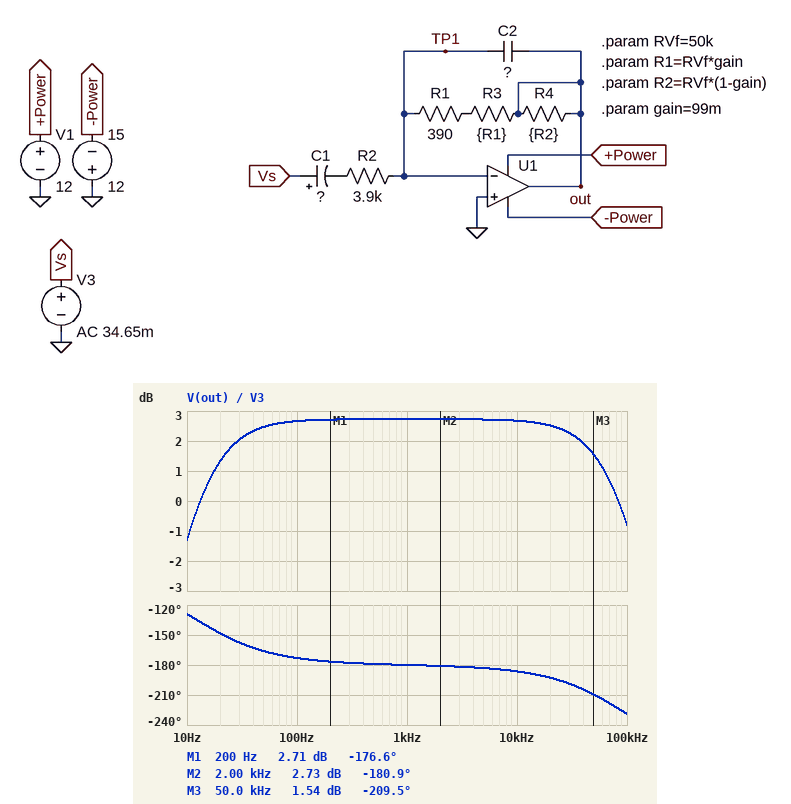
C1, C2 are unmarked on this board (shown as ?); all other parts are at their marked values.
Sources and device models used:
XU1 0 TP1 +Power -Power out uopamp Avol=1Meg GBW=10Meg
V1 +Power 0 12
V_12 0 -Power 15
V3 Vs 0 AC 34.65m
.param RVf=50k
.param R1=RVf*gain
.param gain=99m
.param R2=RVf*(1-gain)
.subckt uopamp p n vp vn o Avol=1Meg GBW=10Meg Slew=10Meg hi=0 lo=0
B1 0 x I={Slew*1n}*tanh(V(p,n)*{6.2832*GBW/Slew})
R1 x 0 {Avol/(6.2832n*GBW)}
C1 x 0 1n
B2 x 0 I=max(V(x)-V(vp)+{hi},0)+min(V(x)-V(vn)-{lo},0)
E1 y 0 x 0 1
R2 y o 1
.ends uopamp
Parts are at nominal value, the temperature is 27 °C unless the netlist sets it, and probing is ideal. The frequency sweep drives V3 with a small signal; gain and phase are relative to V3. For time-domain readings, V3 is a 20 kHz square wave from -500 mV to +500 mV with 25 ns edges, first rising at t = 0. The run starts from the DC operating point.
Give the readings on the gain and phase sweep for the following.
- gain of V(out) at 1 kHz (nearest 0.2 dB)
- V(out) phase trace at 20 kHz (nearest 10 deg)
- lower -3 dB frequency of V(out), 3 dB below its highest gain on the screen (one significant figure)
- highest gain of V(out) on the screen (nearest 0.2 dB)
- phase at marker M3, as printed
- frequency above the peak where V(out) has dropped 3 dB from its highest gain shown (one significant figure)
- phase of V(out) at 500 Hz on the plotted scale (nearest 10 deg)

2.8 dB
-190 deg
10 Hz
2.8 dB
-209.5 deg
90 kHz
-180 deg
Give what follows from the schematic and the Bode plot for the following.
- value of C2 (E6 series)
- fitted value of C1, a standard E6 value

330 pF
3.3 µF
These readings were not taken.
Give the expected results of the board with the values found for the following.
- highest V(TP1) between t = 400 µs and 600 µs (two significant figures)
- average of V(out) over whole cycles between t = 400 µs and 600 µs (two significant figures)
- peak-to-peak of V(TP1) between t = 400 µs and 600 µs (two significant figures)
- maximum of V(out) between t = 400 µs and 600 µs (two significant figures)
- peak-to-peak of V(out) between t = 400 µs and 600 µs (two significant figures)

12 mV
-660 mV
24 mV
31 mV
1.4 V
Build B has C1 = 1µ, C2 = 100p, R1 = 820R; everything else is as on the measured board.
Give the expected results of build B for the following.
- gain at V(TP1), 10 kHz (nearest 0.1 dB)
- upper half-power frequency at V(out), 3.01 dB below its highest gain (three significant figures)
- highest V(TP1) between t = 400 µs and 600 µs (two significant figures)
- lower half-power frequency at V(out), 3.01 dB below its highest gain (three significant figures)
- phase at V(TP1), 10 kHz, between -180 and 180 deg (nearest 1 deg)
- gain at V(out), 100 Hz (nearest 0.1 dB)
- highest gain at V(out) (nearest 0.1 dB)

-56.6 dB
265 kHz
36 mV
40.8 Hz
88 deg
2.7 dB
3.4 dB
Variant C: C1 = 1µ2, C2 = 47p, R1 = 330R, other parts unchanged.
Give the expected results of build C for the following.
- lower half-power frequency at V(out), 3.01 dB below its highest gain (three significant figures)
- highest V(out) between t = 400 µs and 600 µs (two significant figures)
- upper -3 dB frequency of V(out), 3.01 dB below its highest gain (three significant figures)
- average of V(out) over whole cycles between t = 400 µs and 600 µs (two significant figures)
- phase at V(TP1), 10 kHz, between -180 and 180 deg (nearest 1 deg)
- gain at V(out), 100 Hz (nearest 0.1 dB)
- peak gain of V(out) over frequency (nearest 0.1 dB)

34.0 Hz
82 mV
586 kHz
-610 mV
89 deg
2.2 dB
2.6 dB
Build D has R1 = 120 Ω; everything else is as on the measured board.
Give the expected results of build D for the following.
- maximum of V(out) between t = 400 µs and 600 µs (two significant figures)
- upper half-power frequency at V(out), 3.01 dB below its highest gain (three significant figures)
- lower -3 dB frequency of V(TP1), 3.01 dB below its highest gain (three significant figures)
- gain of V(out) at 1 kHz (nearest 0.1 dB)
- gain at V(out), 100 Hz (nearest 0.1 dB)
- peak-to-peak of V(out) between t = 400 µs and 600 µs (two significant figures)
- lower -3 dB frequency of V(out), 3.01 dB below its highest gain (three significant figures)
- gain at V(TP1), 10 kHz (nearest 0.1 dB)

30 mV
94.0 kHz
92.3 kHz
2.3 dB
2.2 dB
1.3 V
12.4 Hz
-57.8 dB
